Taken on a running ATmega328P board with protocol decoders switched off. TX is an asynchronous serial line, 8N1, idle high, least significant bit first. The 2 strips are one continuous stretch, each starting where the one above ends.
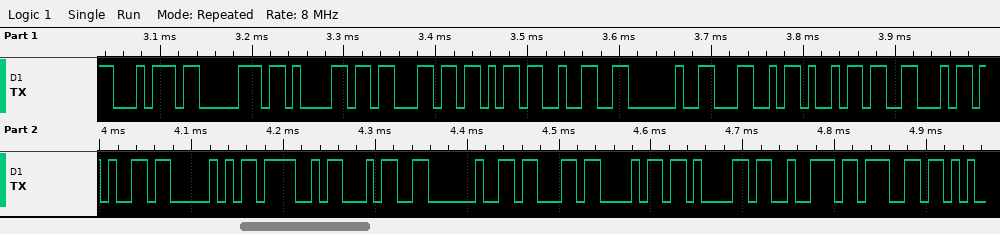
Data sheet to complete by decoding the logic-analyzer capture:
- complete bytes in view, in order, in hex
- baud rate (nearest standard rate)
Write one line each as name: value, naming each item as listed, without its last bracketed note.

complete bytes in view, in order, in hex: 74 70 61 63 6B 32 20 4C 69 46 65 50 4F 34 20 63 68 61 72 67
baud rate: 115200 baud
